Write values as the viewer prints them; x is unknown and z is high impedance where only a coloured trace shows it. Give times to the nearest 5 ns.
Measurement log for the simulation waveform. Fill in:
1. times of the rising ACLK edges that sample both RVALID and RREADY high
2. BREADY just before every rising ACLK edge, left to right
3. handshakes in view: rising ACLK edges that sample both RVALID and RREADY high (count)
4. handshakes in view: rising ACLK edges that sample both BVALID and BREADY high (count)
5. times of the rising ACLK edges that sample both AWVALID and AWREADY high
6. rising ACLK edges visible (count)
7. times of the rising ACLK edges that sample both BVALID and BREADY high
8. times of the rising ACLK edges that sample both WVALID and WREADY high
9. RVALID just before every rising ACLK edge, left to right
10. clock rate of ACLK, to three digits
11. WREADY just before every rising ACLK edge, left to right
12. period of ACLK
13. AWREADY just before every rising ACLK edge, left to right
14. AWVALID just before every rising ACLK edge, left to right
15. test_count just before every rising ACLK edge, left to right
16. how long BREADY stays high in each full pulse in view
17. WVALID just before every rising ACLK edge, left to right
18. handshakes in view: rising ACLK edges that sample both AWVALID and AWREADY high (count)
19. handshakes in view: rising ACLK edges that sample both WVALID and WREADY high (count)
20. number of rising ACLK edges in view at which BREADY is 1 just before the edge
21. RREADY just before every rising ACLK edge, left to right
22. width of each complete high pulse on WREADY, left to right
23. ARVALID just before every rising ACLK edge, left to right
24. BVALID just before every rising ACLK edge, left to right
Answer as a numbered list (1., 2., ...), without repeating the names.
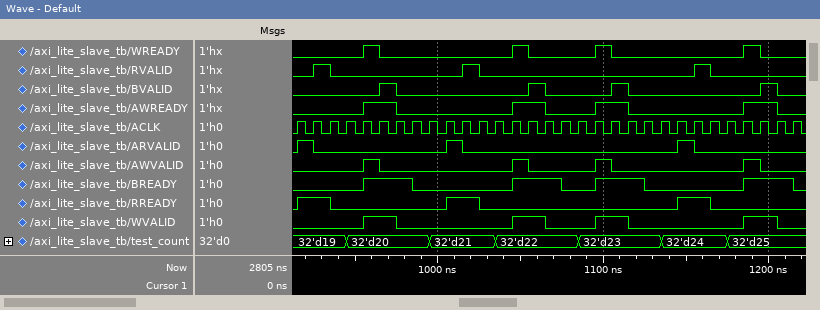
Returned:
1. 935 ns, 1025 ns, 1165 ns
2. 0 0 0 0 0 1 1 1 0 0 0 0 0 0 1 1 1 0 0 1 1 1 0 0 0 0 0 0 1 1 1
3. 3
4. 4
5. 965 ns, 1055 ns, 1105 ns, 1195 ns
6. 31
7. 975 ns, 1065 ns, 1115 ns, 1205 ns
8. 965 ns, 1055 ns, 1105 ns, 1195 ns
9. 0 0 1 0 0 0 0 0 0 0 0 1 0 0 0 0 0 0 0 0 0 0 0 0 0 1 0 0 0 0 0
10. 100 MHz
11. 0 0 0 0 0 1 0 0 0 0 0 0 0 0 1 0 0 0 0 1 0 0 0 0 0 0 0 0 1 0 0
12. 10 ns
13. 0 0 0 0 0 1 1 0 0 0 0 0 0 0 1 1 0 0 0 1 1 0 0 0 0 0 0 0 1 1 0
14. 0 0 0 0 0 1 0 0 0 0 0 0 0 0 1 0 0 0 0 1 0 0 0 0 0 0 0 0 1 0 0
15. 32'd19, 32'd19, 32'd19, 32'd19, 32'd20, 32'd20, 32'd20, 32'd20, 32'd20, 32'd21, 32'd21, 32'd21, 32'd21, 32'd22, 32'd22, 32'd22, 32'd22, 32'd22, 32'd23, 32'd23, 32'd23, 32'd23, 32'd23, 32'd24, 32'd24, 32'd24, 32'd24, 32'd25, 32'd25, 32'd25, 32'd25
16. 30 ns, 30 ns, 30 ns, 30 ns
17. 0 0 0 0 0 1 1 0 0 0 0 0 0 0 1 1 0 0 0 1 1 0 0 0 0 0 0 0 1 1 0
18. 4
19. 4
20. 12
21. 0 1 1 0 0 0 0 0 0 0 1 1 0 0 0 0 0 0 0 0 0 0 0 0 1 1 0 0 0 0 0
22. 10 ns, 10 ns, 10 ns, 10 ns
23. 0 1 0 0 0 0 0 0 0 0 1 0 0 0 0 0 0 0 0 0 0 0 0 0 1 0 0 0 0 0 0
24. 0 0 0 0 0 0 1 0 0 0 0 0 0 0 0 1 0 0 0 0 1 0 0 0 0 0 0 0 0 1 0
